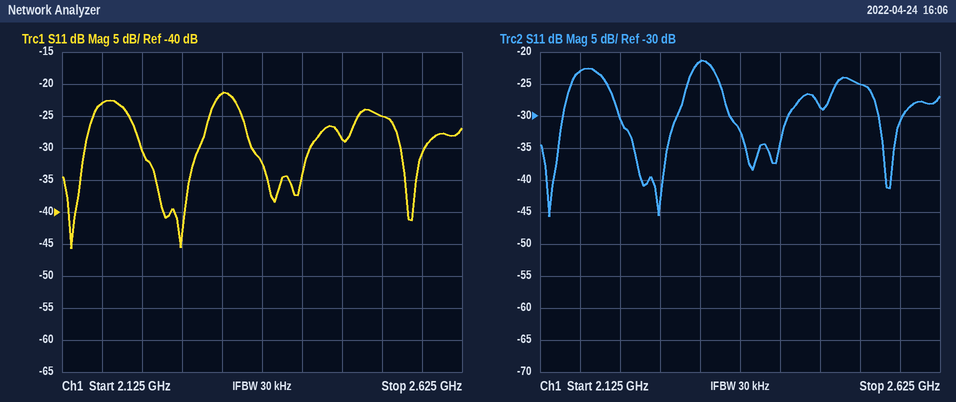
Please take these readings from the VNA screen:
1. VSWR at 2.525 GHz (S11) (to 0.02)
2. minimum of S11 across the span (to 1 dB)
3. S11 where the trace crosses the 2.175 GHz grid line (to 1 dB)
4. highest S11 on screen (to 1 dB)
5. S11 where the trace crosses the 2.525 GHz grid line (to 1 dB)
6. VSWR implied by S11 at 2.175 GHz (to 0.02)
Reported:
1.12
-46 dB
-23 dB
-21 dB
-25 dB
1.16
